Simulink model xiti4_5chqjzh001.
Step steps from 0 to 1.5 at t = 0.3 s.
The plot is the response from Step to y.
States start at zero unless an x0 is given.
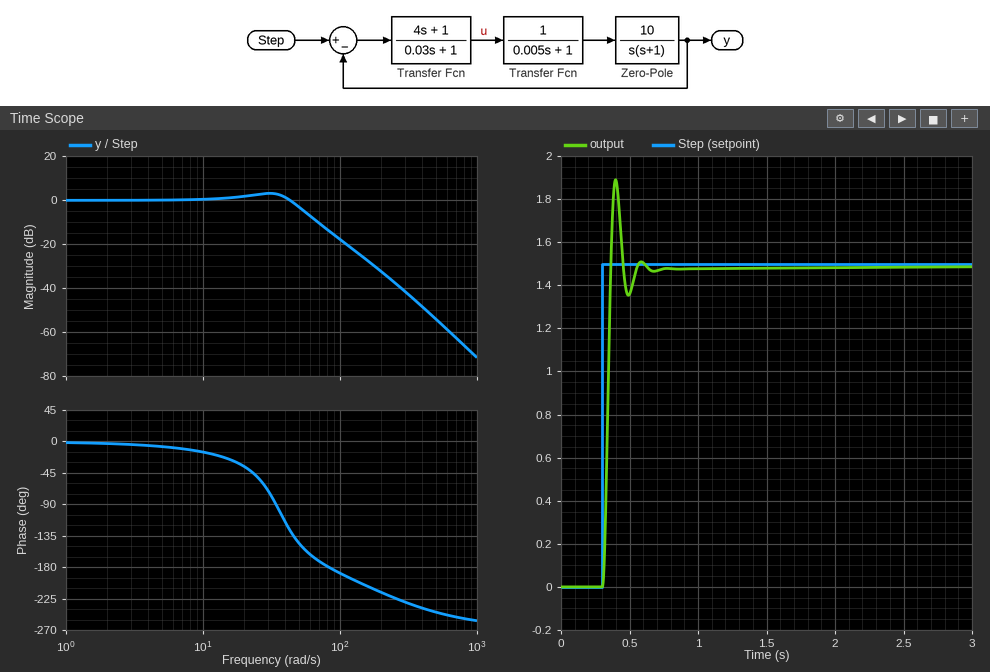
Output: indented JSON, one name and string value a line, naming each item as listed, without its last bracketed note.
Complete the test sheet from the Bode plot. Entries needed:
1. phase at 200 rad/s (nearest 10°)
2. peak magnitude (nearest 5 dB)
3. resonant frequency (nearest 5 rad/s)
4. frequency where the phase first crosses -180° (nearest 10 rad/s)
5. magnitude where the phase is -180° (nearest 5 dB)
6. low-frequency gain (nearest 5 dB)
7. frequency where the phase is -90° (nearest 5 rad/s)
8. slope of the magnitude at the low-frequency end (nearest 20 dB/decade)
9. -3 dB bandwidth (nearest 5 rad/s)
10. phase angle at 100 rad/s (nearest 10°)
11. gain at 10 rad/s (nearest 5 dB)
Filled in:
{
  "phase at 200 rad/s": "-220°",
  "peak magnitude": "5 dB",
  "resonant frequency": "30 rad/s",
  "frequency where the phase first crosses -180°": "80 rad/s",
  "magnitude where the phase is -180°": "-15 dB",
  "low-frequency gain": "0 dB",
  "frequency where the phase is -90°": "35 rad/s",
  "slope of the magnitude at the low-frequency end": "0 dB/decade",
  "-3 dB bandwidth": "50 rad/s",
  "phase angle at 100 rad/s": "-190°",
  "gain at 10 rad/s": "0 dB"
}
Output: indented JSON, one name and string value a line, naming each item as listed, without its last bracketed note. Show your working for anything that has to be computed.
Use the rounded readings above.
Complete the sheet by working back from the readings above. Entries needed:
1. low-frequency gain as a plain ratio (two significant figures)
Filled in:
{
  "low-frequency gain as a plain ratio": "10^(0 / 20) = 1.0"
}
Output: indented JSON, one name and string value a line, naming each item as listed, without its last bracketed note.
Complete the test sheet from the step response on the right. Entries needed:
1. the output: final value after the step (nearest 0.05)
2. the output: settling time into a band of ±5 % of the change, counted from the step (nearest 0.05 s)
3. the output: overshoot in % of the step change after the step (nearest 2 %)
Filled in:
{
  "the output: final value after the step": "1.50",
  "the output: settling time into a band of ±5 % of the change, counted from the step": "0.25 s",
  "the output: overshoot in % of the step change after the step": "26 %"
}
